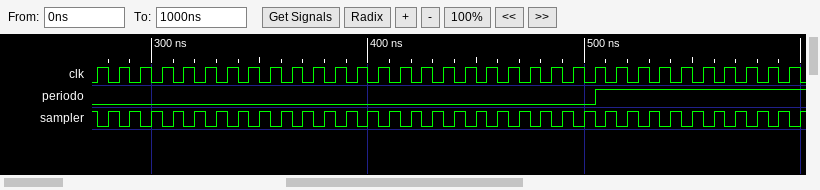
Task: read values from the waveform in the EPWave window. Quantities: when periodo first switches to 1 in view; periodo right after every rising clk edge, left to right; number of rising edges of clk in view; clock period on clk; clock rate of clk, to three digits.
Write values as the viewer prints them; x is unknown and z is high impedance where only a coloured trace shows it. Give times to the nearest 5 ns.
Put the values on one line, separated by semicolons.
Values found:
505 ns; 0 0 0 0 0 0 0 0 0 0 0 0 0 0 0 0 0 0 0 0 0 0 0 1 1 1 1 1 1 1 1 1 1; 33; 10 ns; 100 MHz
